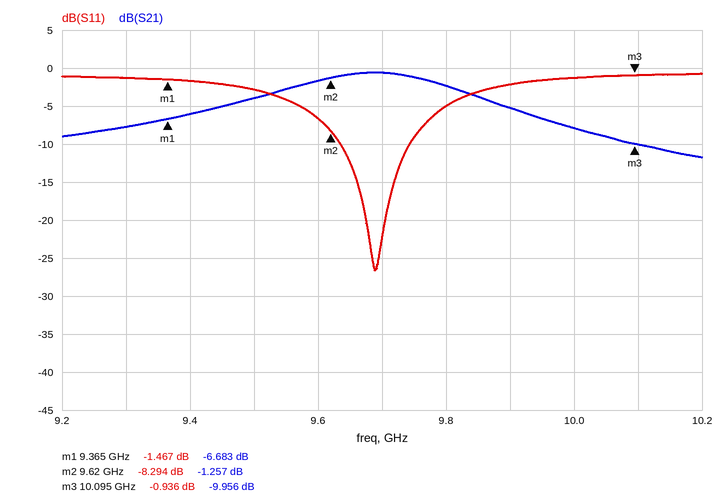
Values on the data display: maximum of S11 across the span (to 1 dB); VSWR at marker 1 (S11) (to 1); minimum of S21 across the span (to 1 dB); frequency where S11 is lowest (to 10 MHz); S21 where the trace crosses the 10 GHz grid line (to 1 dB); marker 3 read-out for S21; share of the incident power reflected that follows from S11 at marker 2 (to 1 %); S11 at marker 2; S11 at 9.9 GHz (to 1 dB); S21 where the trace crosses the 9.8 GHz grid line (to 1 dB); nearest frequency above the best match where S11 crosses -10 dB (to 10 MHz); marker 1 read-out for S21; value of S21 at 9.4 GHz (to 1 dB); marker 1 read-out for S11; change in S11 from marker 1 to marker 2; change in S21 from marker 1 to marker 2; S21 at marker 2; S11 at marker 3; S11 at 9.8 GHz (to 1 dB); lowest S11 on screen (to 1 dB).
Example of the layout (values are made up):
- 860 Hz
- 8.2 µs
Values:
- -1 dB
- 12
- -12 dB
- 9.69 GHz
- -8 dB
- -9.956 dB
- 15 %
- -8.294 dB
- -2 dB
- -2 dB
- 9.74 GHz
- -6.683 dB
- -6 dB
- -1.467 dB
- -6.827 dB
- 5.426 dB
- -1.257 dB
- -0.936 dB
- -5 dB
- -27 dB
